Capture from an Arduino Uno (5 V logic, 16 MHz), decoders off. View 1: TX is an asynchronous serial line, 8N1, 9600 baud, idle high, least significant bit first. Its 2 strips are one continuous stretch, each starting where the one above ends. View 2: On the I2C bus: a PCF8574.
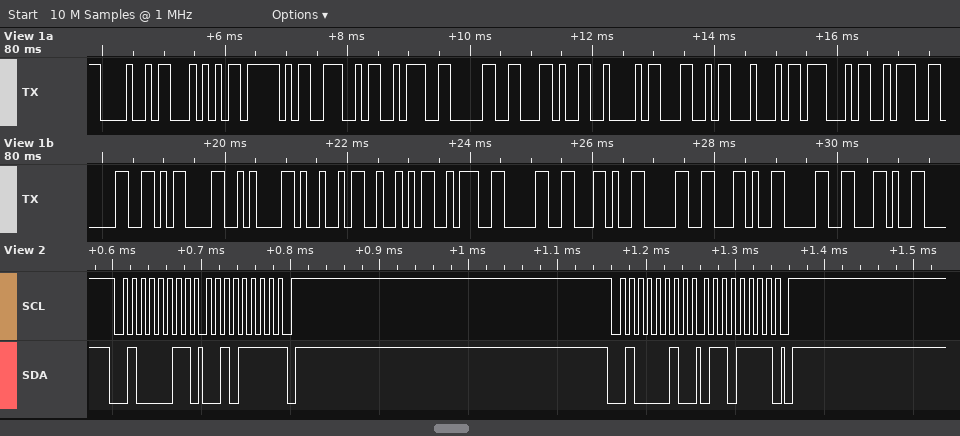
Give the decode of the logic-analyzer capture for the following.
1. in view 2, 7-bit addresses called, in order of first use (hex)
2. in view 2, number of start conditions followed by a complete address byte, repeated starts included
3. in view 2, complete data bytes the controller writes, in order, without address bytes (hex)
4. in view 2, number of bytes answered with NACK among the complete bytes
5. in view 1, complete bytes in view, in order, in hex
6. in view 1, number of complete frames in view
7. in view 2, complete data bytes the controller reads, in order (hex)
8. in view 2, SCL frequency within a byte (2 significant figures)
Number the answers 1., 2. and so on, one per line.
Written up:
1. 0x21
2. 2
3. 6F
4. 1
5. 48 54 5F 4E 3A 30 2C 42 4C 44 47 3A 30 0D 0A 49 52 3A 30 2C 30 2C 30 2C
6. 24
7. 2F
8. 100 kHz
